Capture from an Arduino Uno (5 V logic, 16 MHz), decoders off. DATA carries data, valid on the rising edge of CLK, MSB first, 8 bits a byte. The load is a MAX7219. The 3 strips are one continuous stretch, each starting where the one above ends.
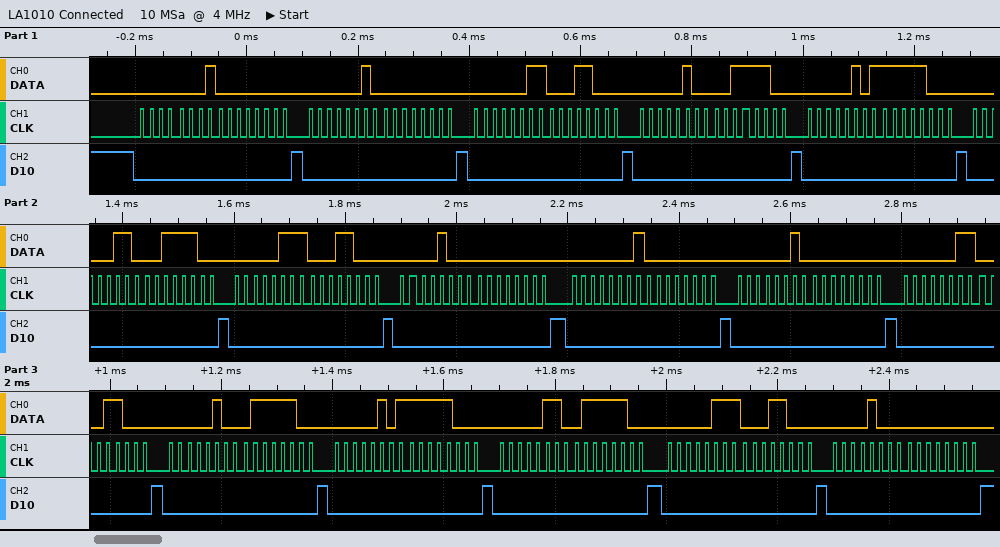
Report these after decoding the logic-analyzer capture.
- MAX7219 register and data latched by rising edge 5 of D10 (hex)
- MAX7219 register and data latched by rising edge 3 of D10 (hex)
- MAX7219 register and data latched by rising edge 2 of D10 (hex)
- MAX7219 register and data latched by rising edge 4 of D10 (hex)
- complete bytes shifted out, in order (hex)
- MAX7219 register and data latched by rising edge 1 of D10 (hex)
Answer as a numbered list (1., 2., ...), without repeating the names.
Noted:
1. register 0x5, data 0xF8
2. register 0x3, data 0x18
3. register 0x2, data 0x00
4. register 0x4, data 0x3C
5. 01 00 02 00 03 18 04 3C 05 F8 06 3C 07 18 08 00 01 00 02 00 03 18 04 7C 05 F8 06 7C 07 18 08 00
6. register 0x1, data 0x00
